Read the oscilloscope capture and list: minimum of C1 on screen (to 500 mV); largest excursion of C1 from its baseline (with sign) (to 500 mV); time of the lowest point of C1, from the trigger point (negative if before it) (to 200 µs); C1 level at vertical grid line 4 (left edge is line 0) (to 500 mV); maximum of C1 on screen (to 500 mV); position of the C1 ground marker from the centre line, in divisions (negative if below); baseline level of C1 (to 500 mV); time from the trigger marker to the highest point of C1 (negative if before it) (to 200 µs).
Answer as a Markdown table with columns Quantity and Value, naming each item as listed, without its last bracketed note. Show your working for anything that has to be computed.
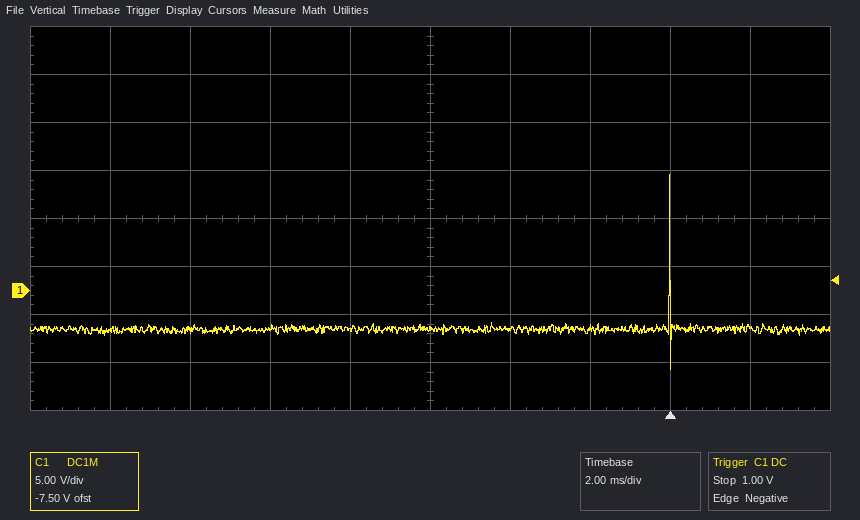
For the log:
| Quantity | Value |
|---|---|
| minimum of C1 on screen | -8.0 V |
| largest excursion of C1 from its baseline (with sign) | 12.0 V − (-4.0 V) = +16.0 V |
| time of the lowest point of C1, from the trigger point (negative if before it) | 0.0 ms |
| C1 level at vertical grid line 4 (left edge is line 0) | -4.0 V |
| maximum of C1 on screen | 12.0 V |
| position of the C1 ground marker from the centre line, in divisions | -1.5 div |
| baseline level of C1 | -4.0 V |
| time from the trigger marker to the highest point of C1 (negative if before it) | 0.0 ms |
